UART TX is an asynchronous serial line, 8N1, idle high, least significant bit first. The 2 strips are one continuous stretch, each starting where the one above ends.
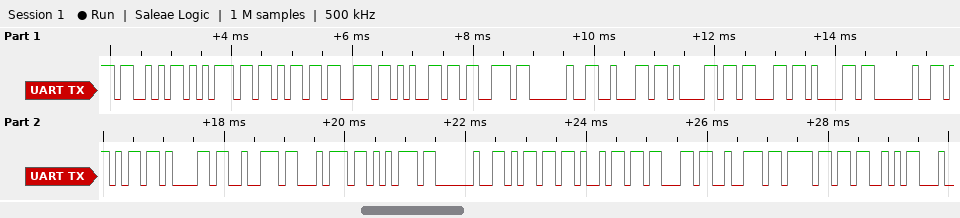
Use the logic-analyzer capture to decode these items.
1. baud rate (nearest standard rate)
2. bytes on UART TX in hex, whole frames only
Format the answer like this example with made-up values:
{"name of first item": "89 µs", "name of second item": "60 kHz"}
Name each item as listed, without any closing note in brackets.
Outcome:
{"baud rate": "9600 baud", "bytes on UART TX in hex, whole frames only": "0x53 0x75 0x6B 0x73 0x65 0x73 0x20 0x62 0x61 0x63 0x61 0x20 0x6B 0x61 0x72 0x74 0x75 0x20 0x6D 0x69 0x63 0x72 0x6F 0x53"}
